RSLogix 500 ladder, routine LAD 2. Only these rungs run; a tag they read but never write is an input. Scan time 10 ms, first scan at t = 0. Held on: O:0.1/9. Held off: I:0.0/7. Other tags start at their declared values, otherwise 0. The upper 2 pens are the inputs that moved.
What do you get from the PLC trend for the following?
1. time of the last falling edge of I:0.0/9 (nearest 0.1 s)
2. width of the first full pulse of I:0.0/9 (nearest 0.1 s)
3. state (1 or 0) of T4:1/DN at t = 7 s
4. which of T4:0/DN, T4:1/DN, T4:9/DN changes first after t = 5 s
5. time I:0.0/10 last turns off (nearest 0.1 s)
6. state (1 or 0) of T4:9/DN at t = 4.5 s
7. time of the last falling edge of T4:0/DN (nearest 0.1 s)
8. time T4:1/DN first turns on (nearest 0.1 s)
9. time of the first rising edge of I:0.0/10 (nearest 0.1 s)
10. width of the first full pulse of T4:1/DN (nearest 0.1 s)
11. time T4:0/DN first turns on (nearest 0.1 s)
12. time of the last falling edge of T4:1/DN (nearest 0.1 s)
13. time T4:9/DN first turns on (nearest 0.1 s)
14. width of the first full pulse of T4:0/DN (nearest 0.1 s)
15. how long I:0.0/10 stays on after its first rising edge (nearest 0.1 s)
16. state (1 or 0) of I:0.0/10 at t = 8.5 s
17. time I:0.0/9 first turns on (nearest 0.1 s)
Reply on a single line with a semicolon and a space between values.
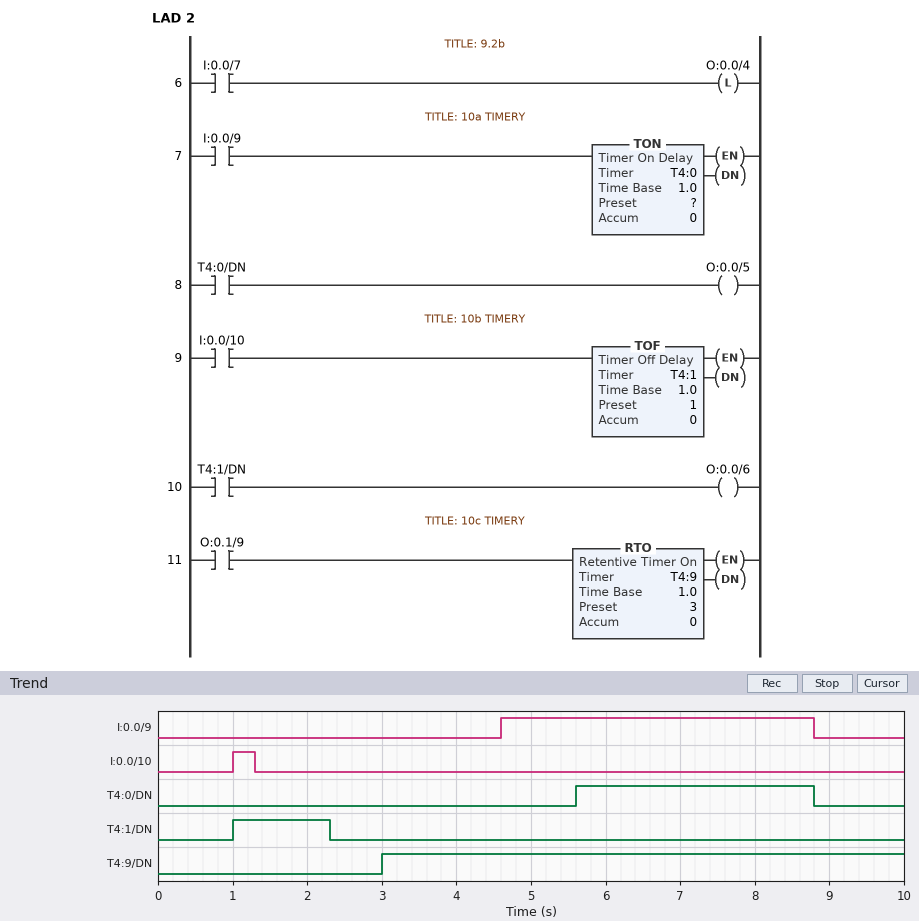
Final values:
8.8 s; 4.2 s; 0; T4:0/DN; 1.3 s; 1; 8.8 s; 1.0 s; 1.0 s; 1.3 s; 5.6 s; 2.3 s; 3.0 s; 3.2 s; 0.3 s; 0; 4.6 s
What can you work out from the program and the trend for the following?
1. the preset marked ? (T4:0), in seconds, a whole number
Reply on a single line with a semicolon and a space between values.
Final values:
1 s
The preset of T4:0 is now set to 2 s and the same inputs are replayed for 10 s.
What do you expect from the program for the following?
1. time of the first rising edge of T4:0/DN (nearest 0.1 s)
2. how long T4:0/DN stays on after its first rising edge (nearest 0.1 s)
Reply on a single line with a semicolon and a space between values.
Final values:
6.6 s; 2.2 s
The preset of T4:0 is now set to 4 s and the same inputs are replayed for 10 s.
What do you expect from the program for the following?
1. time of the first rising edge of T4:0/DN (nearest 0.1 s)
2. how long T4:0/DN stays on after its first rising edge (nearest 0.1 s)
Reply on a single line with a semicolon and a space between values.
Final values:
8.6 s; 0.2 s
